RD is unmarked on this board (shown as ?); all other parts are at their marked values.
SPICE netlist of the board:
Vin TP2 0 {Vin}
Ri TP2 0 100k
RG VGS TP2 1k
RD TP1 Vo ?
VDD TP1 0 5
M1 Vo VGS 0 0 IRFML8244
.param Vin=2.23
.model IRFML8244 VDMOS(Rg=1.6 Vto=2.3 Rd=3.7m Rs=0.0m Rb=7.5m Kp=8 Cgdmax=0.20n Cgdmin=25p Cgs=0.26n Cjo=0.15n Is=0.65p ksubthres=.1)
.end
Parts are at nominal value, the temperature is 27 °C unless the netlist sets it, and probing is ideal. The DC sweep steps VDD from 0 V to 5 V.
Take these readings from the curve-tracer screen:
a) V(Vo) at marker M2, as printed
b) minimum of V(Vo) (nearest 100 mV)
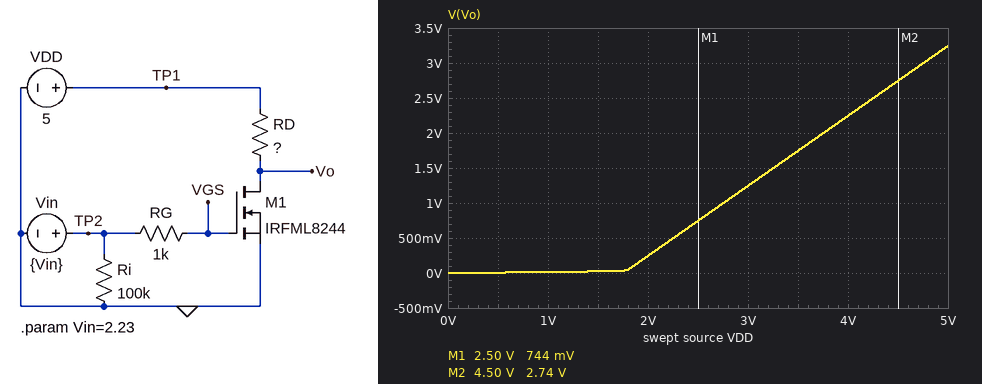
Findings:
2.74 V
0 V
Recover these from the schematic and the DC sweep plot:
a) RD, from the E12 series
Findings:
270 Ω
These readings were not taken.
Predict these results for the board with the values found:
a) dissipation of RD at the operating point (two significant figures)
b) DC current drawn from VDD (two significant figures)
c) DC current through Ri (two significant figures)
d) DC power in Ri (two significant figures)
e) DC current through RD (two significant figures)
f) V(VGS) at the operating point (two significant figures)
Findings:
11 mW
6.5 mA
22 µA
50 µW
6.5 mA
2.2 V
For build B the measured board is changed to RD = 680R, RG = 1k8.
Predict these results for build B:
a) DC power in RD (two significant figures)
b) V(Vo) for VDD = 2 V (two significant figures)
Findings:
29 mW
10 mV
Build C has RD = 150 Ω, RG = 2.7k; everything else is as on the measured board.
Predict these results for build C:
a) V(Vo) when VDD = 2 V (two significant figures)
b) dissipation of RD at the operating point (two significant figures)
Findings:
1.0 V
6.3 mW
